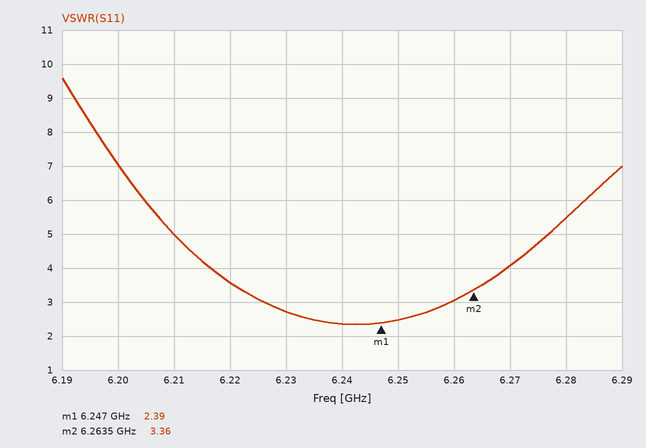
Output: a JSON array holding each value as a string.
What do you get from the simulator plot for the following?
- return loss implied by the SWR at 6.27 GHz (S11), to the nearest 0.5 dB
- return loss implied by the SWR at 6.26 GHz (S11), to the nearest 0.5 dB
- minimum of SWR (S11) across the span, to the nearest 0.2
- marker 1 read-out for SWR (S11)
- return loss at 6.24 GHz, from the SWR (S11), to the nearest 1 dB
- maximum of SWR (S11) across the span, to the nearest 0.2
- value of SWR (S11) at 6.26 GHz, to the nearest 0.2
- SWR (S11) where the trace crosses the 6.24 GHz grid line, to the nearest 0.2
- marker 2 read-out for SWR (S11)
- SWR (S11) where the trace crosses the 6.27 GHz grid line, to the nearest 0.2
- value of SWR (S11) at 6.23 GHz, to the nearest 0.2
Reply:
["4.5 dB", "6.0 dB", "2.4", "2.39", "8 dB", "9.6", "3.0", "2.4", "3.36", "4.0", "2.8"]
